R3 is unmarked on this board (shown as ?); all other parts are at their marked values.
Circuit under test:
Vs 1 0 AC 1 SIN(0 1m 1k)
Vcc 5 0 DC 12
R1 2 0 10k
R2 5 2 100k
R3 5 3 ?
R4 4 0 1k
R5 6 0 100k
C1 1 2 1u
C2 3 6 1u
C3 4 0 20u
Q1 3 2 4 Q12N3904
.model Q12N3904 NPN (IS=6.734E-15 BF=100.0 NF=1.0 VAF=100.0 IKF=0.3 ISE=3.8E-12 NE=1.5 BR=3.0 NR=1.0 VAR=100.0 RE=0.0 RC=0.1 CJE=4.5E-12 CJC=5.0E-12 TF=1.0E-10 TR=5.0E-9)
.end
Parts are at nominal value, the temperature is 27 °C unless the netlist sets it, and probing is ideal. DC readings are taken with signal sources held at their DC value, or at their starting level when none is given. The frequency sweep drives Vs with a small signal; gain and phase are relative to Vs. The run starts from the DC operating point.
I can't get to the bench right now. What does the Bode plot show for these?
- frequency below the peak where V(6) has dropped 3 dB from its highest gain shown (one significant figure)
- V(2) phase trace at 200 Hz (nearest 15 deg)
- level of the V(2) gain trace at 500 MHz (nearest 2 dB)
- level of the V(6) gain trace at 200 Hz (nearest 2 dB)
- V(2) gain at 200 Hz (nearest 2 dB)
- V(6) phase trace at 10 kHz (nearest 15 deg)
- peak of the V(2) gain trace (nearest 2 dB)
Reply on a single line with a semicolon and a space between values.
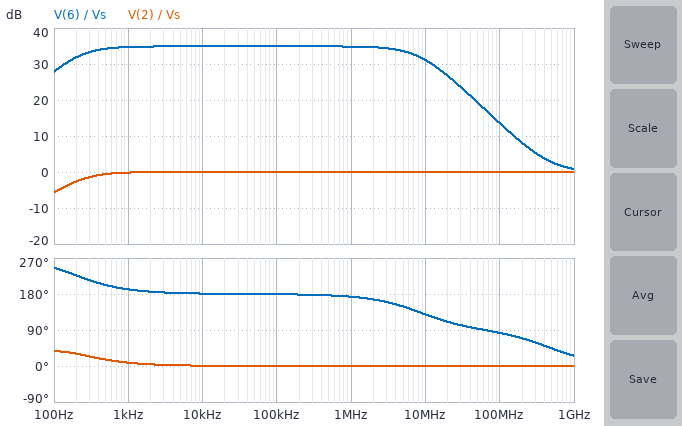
200 Hz; 30 deg; 0 dB; 32 dB; -2 dB; 180 deg; 0 dB
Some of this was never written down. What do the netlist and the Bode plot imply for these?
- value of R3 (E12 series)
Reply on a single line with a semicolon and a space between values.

10 kΩ
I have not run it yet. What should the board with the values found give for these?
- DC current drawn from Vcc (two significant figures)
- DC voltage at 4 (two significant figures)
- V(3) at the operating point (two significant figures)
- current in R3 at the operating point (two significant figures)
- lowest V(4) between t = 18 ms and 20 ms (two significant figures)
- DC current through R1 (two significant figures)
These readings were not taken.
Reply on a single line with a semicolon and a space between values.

270 µA; 190 mV; 10 V; 160 µA; 190 mV; 81 µA
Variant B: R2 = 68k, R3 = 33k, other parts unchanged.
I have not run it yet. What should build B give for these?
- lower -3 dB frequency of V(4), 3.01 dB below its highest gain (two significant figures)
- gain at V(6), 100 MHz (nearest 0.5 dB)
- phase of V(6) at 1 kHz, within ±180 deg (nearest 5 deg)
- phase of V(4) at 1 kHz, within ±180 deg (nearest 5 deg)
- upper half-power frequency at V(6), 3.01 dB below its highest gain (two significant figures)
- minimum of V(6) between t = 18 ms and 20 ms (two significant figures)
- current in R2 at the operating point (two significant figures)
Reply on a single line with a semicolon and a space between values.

9.3 Hz; 10.0 dB; -150 deg; -60 deg; 2.0 MHz; -67 mV; 160 µA
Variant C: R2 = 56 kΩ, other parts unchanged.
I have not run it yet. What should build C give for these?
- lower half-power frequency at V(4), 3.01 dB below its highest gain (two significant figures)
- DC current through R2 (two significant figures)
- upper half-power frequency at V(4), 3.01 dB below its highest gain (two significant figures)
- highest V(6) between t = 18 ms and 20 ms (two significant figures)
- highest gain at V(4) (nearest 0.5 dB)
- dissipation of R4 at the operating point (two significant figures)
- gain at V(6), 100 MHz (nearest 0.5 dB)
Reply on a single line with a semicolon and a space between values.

11 Hz; 190 µA; 500 Hz; 150 mV; -9.5 dB; 330 µW; 22.0 dB
